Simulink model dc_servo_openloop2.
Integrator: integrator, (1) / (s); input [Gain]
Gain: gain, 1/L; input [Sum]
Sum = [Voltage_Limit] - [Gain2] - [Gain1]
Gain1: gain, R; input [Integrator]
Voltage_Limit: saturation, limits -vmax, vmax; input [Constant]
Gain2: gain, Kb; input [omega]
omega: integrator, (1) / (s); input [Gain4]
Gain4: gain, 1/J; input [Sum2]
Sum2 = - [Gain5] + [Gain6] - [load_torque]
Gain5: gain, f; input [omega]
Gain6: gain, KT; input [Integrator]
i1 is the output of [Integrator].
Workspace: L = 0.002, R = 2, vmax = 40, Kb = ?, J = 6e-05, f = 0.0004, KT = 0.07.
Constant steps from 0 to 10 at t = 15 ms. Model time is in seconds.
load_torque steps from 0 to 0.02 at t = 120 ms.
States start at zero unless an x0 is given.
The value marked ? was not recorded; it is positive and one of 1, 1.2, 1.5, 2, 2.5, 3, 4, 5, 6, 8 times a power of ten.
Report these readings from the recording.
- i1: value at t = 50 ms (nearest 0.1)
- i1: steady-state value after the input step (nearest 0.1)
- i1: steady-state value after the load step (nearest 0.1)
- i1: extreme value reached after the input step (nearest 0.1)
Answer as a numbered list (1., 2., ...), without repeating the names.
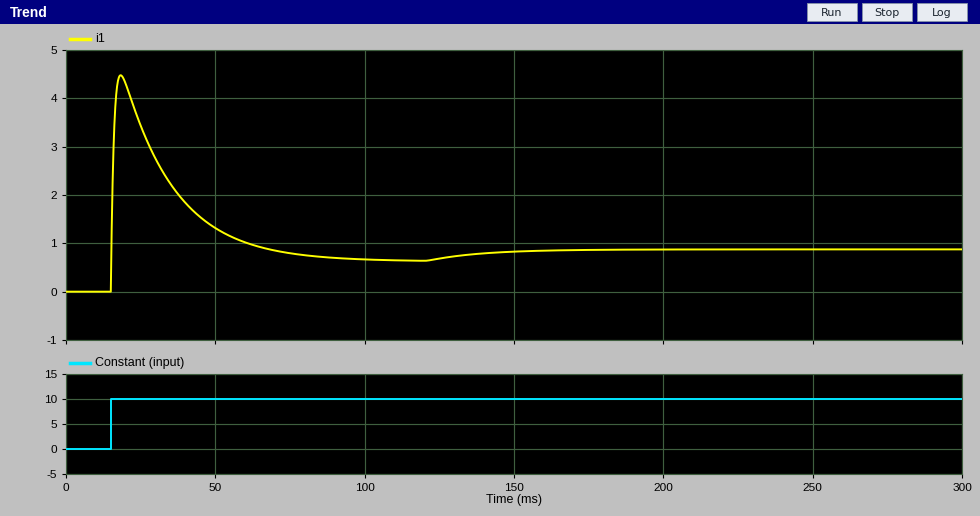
1. 1.3
2. 0.6
3. 0.9
4. 4.5
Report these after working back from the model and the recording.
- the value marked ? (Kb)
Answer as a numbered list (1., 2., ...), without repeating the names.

1. 0.08
